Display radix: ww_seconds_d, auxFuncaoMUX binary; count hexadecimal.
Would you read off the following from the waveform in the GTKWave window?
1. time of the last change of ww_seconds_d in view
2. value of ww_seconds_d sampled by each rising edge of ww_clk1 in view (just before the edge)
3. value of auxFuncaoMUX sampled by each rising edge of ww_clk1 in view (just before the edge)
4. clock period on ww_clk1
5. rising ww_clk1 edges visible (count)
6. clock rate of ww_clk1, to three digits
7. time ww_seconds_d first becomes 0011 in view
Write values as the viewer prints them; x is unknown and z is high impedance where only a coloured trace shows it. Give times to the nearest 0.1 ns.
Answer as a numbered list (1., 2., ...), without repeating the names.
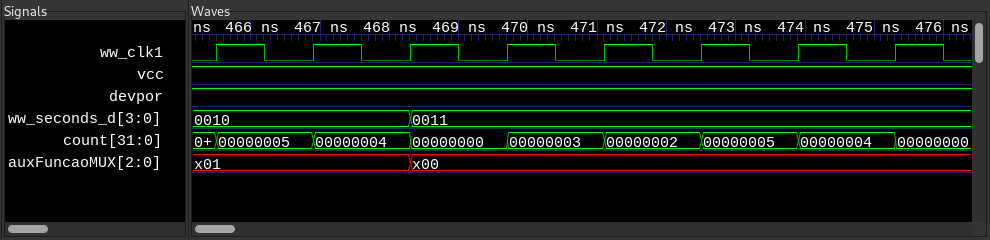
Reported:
1. 468.3 ns
2. 0010, 0010, 0010, 0011, 0011, 0011, 0011, 0011
3. x01, x01, x01, x00, x00, x00, x00, x00
4. 1.4 ns
5. 8
6. 714 MHz
7. 468.3 ns
